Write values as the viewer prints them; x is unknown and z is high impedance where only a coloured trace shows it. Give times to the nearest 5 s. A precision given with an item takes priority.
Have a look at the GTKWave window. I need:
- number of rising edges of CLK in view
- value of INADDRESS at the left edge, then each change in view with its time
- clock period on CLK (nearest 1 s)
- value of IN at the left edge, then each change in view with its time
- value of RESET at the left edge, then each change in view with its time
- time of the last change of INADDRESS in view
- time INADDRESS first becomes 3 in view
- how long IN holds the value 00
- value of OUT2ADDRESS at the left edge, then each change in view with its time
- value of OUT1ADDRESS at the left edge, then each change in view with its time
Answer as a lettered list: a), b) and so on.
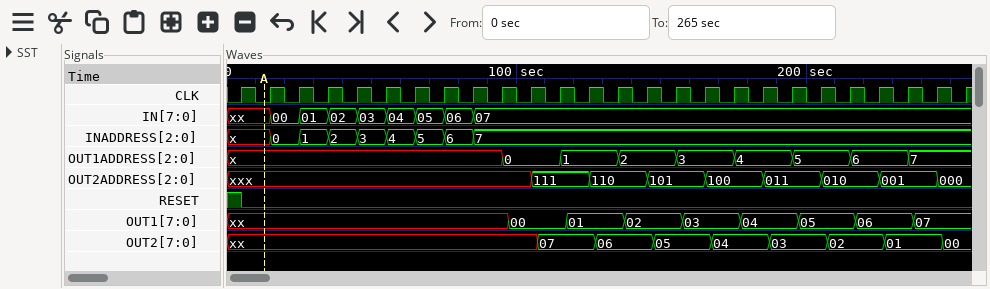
a) 26
b) x, 0 at 15 s, 1 at 25 s, 2 at 35 s, 3 at 45 s, 4 at 55 s, 5 at 65 s, 6 at 75 s, 7 at 85 s
c) 10 s
d) xx, 00 at 15 s, 01 at 25 s, 02 at 35 s, 03 at 45 s, 04 at 55 s, 05 at 65 s, 06 at 75 s, 07 at 85 s
e) 1, 0 at 5 s
f) 85 s
g) 45 s
h) 10 s
i) xxx, 111 at 105 s, 110 at 125 s, 101 at 145 s, 100 at 165 s, 011 at 185 s, 010 at 205 s, 001 at 225 s, 000 at 245 s
j) x, 0 at 95 s, 1 at 115 s, 2 at 135 s, 3 at 155 s, 4 at 175 s, 5 at 195 s, 6 at 215 s, 7 at 235 s
